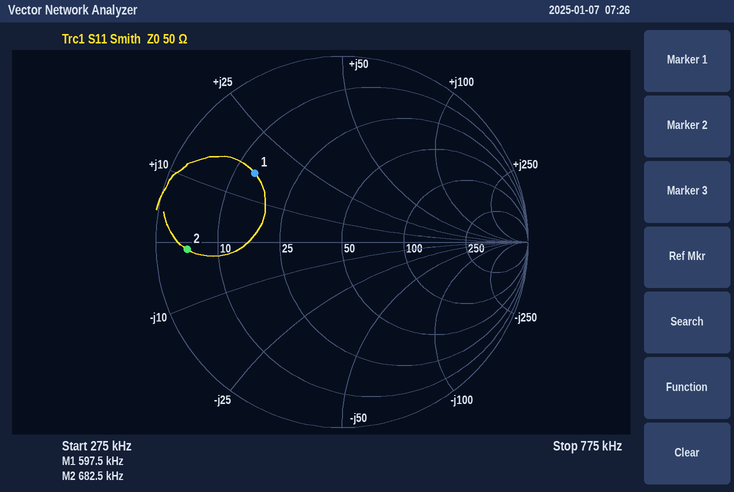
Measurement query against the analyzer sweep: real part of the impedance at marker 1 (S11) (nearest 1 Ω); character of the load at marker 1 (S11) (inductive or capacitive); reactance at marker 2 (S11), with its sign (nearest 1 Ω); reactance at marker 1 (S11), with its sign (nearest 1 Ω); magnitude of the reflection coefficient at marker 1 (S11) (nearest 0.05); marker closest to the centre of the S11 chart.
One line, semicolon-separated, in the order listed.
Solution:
14 Ω; inductive; -1 Ω; +16 Ω; 0.60; marker 1
